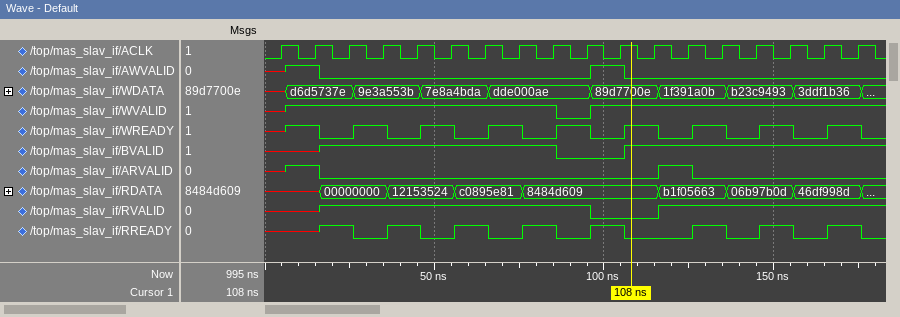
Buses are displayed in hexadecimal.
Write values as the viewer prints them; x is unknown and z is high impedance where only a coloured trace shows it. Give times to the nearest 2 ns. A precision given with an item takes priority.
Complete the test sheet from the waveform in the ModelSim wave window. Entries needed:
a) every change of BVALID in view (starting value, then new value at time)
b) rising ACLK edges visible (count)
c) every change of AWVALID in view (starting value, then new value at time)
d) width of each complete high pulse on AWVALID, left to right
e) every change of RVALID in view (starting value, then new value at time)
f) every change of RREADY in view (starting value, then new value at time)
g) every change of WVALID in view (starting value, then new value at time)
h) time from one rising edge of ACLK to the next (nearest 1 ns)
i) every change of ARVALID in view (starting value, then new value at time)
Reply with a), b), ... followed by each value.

a) x, 1 at 16 ns, 0 at 86 ns, 1 at 106 ns
b) 18
c) x, 1 at 6 ns, 0 at 16 ns, 1 at 96 ns, 0 at 106 ns
d) 10 ns
e) x, 1 at 16 ns, 0 at 96 ns, 1 at 116 ns
f) x, 1 at 16 ns, 0 at 26 ns, 1 at 36 ns, 0 at 46 ns, 1 at 56 ns, 0 at 66 ns, 1 at 76 ns, 0 at 86 ns, 1 at 96 ns, 0 at 106 ns, 1 at 126 ns, 0 at 136 ns, 1 at 146 ns, 0 at 156 ns, 1 at 166 ns, 0 at 176 ns
g) x, 1 at 6 ns, 0 at 86 ns, 1 at 96 ns
h) 10 ns
i) x, 1 at 6 ns, 0 at 16 ns, 1 at 116 ns, 0 at 126 ns
